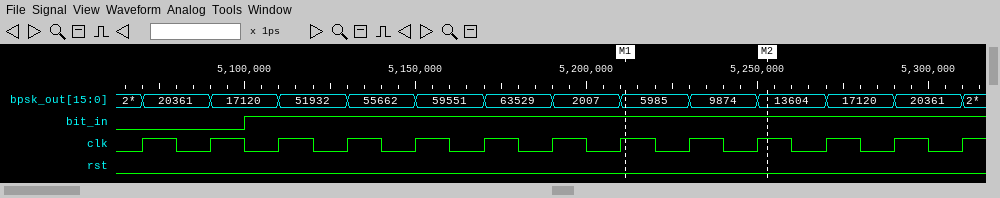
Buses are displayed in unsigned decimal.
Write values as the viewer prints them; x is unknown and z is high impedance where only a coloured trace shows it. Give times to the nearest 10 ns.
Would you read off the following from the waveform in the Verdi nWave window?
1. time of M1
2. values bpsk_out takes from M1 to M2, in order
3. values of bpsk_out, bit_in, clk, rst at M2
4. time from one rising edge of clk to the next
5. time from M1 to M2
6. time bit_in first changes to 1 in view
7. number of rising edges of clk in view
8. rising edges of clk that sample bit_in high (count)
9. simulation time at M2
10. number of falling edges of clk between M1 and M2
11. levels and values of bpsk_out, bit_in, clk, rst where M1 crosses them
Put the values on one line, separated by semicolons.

5210 ns; 5985, 9874, 13604; bpsk_out=13604, bit_in=1, clk=1, rst=0; 20 ns; 40 ns; 5100 ns; 13; 11; 5250 ns; 2; bpsk_out=5985, bit_in=1, clk=1, rst=0
